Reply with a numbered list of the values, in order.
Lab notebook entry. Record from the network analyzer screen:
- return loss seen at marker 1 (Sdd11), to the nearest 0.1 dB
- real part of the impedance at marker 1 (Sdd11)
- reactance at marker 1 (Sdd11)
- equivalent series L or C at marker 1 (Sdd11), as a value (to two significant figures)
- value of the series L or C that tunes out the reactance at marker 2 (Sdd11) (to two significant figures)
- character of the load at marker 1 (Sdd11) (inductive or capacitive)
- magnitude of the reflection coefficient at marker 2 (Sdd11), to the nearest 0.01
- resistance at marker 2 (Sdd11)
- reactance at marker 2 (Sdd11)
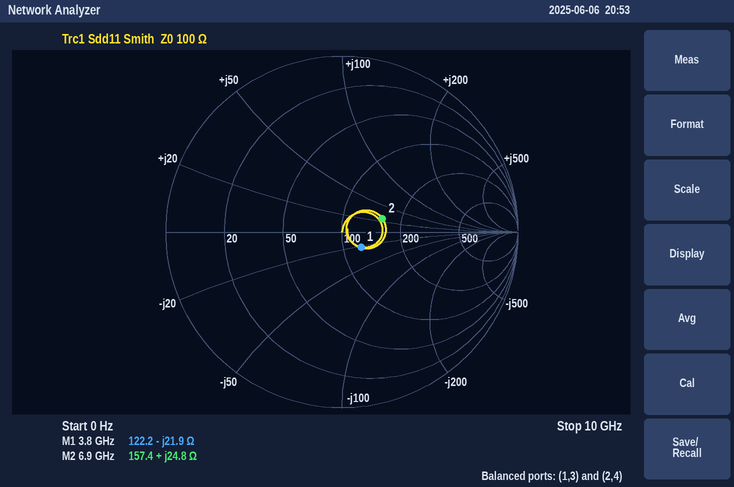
1. 17.1 dB
2. 122.2 Ω
3. -21.9 Ω
4. 1.9 pF
5. 930 fF
6. capacitive
7. 0.24
8. 157.4 Ω
9. +24.8 Ω
